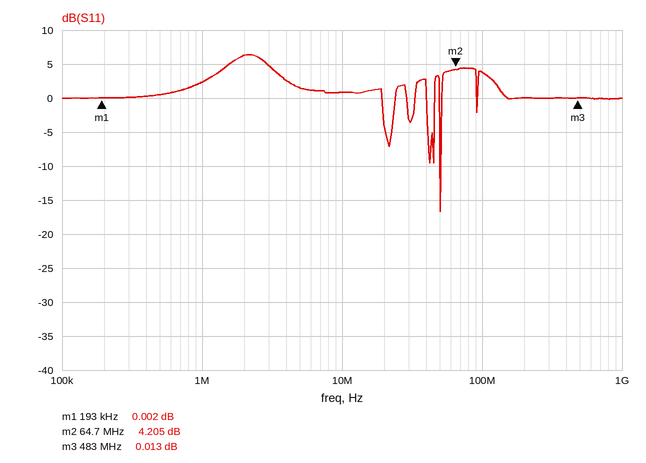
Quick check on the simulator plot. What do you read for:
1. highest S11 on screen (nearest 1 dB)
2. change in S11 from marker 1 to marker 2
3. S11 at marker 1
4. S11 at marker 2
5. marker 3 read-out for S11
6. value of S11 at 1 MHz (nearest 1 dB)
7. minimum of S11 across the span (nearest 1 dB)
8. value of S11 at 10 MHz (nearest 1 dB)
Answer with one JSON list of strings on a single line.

["6 dB", "4.203 dB", "0.002 dB", "4.205 dB", "0.013 dB", "2 dB", "-17 dB", "1 dB"]
